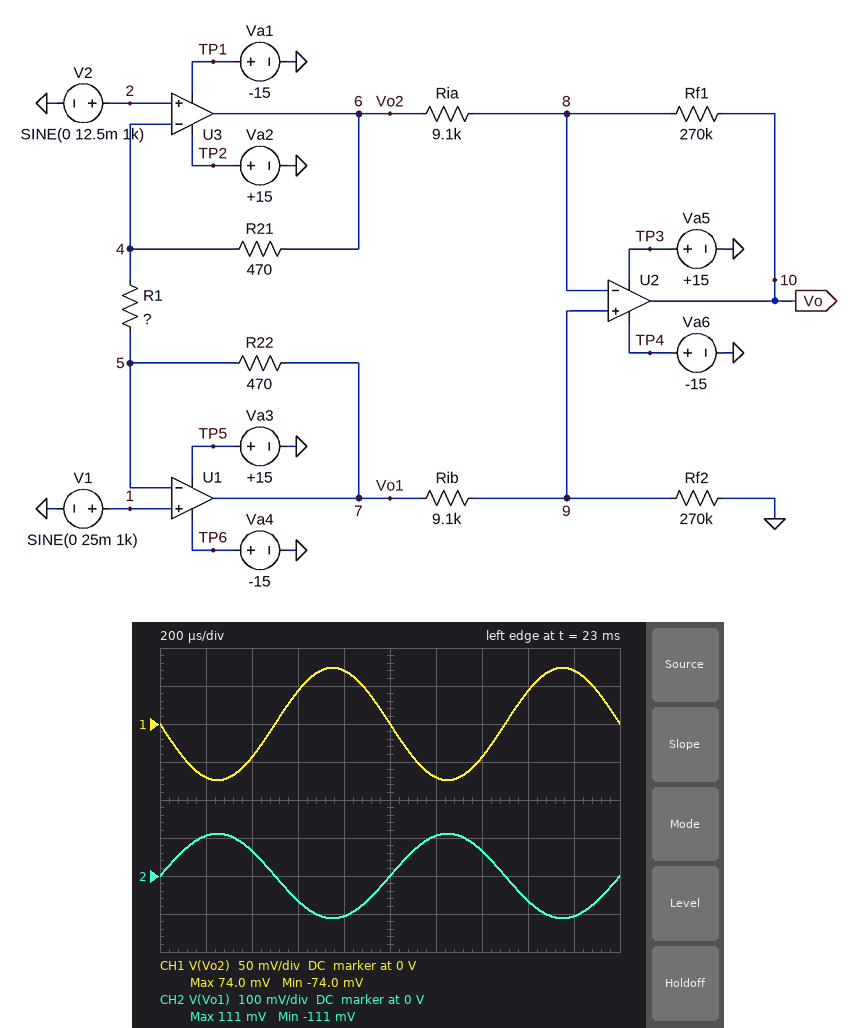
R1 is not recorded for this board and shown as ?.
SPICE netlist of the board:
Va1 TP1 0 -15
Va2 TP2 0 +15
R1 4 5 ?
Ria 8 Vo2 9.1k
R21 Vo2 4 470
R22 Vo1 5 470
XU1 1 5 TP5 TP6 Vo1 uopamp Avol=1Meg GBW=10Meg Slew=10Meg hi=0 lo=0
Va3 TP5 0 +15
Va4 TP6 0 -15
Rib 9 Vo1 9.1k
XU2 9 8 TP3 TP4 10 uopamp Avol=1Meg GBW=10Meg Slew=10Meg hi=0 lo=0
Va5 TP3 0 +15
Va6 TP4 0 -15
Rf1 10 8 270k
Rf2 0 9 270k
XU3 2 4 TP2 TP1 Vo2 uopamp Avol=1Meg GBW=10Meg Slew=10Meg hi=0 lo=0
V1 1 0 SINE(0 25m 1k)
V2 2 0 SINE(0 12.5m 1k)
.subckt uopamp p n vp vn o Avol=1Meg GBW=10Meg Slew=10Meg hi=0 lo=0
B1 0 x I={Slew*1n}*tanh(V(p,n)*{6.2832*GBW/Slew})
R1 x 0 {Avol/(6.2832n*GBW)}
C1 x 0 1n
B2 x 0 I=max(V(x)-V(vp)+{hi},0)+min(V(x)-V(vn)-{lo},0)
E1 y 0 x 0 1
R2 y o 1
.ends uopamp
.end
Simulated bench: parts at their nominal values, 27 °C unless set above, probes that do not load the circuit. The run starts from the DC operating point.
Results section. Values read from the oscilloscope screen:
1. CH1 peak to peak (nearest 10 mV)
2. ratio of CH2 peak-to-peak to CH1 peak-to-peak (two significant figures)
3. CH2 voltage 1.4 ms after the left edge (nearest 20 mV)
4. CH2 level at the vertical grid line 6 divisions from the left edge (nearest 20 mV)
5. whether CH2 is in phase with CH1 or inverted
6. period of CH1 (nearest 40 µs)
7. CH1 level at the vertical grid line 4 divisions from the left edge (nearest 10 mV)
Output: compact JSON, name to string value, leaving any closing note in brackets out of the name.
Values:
{"CH1 peak to peak": "150 mV", "ratio of CH2 peak-to-peak to CH1 peak-to-peak": "1.5", "CH2 voltage 1.4 ms after the left edge": "60 mV", "CH2 level at the vertical grid line 6 divisions from the left edge": "100 mV", "whether CH2 is in phase with CH1 or inverted": "inverted", "period of CH1": "1.00 ms", "CH1 level at the vertical grid line 4 divisions from the left edge": "70 mV"}
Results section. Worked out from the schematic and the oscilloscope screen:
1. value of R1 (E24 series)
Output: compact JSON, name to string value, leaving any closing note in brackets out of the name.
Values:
{"value of R1": "68 Ω"}
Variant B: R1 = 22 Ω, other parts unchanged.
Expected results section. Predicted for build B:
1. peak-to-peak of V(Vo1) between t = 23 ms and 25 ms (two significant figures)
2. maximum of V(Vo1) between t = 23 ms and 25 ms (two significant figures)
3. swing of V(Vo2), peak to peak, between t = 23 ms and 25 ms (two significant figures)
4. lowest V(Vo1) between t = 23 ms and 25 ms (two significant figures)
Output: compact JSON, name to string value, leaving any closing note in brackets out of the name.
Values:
{"peak-to-peak of V(Vo1) between t = 23 ms and 25 ms": "580 mV", "maximum of V(Vo1) between t = 23 ms and 25 ms": "290 mV", "swing of V(Vo2), peak to peak, between t = 23 ms and 25 ms": "510 mV", "lowest V(Vo1) between t = 23 ms and 25 ms": "-290 mV"}
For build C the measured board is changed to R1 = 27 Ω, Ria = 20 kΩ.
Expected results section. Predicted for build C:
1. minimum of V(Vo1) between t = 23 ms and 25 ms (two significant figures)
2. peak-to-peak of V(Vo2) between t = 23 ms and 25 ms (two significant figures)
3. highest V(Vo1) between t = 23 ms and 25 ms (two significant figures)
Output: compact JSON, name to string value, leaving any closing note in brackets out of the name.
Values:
{"minimum of V(Vo1) between t = 23 ms and 25 ms": "-240 mV", "peak-to-peak of V(Vo2) between t = 23 ms and 25 ms": "410 mV", "highest V(Vo1) between t = 23 ms and 25 ms": "240 mV"}
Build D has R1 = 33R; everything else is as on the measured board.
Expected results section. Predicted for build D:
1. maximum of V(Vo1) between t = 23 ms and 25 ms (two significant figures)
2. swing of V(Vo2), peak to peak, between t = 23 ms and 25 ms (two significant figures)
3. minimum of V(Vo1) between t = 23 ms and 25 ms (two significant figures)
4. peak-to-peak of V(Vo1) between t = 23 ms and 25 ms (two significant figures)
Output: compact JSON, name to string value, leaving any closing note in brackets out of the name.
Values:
{"maximum of V(Vo1) between t = 23 ms and 25 ms": "200 mV", "swing of V(Vo2), peak to peak, between t = 23 ms and 25 ms": "330 mV", "minimum of V(Vo1) between t = 23 ms and 25 ms": "-200 mV", "peak-to-peak of V(Vo1) between t = 23 ms and 25 ms": "410 mV"}
